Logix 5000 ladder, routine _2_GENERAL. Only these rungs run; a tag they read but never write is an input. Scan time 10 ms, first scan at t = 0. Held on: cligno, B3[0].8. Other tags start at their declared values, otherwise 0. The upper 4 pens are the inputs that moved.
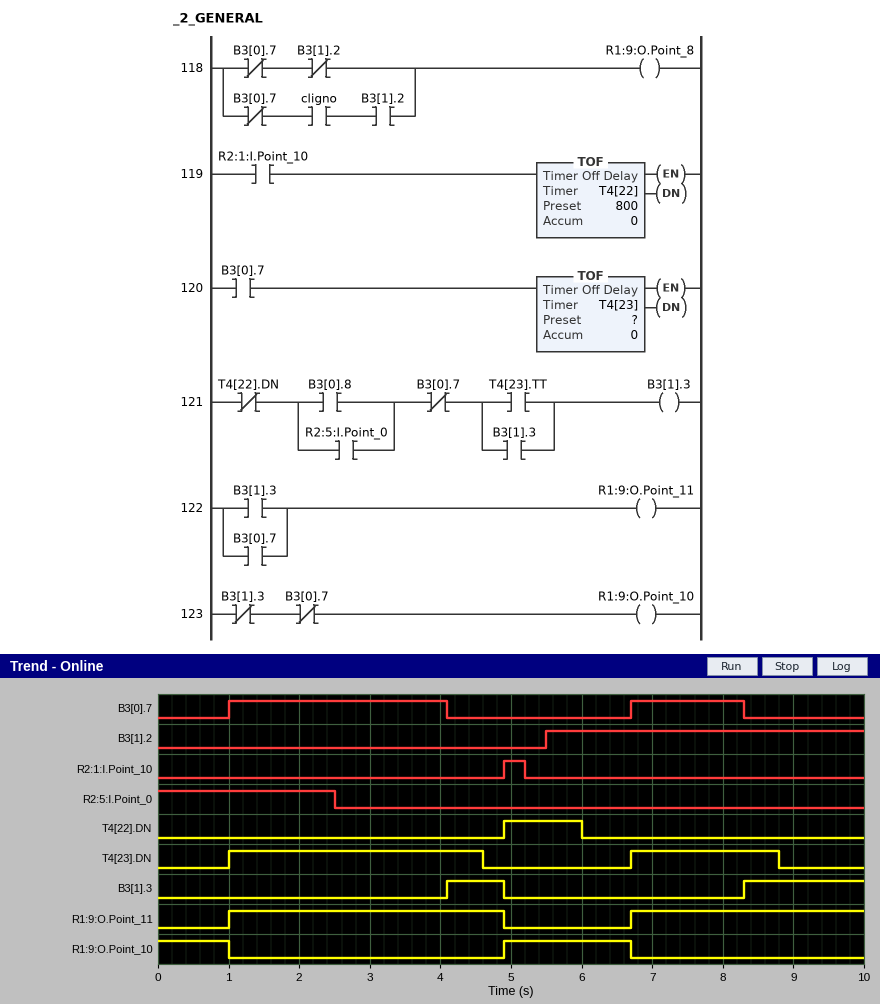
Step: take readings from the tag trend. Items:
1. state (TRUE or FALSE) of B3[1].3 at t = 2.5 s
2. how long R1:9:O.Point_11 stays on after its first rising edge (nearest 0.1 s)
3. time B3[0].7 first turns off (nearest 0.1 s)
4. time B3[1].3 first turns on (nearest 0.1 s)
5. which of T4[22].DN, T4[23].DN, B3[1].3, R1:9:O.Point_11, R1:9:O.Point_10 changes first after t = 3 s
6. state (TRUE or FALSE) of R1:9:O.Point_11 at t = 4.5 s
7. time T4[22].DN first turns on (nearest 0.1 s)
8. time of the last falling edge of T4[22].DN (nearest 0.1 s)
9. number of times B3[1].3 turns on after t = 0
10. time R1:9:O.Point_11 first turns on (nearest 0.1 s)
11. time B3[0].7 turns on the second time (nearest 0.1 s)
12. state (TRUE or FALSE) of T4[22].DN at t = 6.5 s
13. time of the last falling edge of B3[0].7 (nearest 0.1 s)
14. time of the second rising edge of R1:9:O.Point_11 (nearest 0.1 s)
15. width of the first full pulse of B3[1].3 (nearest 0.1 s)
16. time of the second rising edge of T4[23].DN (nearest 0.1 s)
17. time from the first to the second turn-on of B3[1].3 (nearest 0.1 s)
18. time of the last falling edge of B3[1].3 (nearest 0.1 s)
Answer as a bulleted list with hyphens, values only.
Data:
- FALSE
- 3.9 s
- 4.1 s
- 4.1 s
- B3[1].3
- TRUE
- 4.9 s
- 6.0 s
- 2
- 1.0 s
- 6.7 s
- FALSE
- 8.3 s
- 6.7 s
- 0.8 s
- 6.7 s
- 4.2 s
- 4.9 s
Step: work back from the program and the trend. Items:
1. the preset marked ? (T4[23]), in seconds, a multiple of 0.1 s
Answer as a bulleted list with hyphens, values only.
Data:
- 0.5 s
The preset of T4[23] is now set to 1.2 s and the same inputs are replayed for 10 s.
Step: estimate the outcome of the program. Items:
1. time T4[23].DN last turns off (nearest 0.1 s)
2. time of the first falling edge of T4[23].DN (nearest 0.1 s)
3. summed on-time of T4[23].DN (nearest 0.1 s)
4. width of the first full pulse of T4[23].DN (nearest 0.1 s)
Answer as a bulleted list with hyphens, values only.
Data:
- 9.5 s
- 5.3 s
- 7.1 s
- 4.3 s
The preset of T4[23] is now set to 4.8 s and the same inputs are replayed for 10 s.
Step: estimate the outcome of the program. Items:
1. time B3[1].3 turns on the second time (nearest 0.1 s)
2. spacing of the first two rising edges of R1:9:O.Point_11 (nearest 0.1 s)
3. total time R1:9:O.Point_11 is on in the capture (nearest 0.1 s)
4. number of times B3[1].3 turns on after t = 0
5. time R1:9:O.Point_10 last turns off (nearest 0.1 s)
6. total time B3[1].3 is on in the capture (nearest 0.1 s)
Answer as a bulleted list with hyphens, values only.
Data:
- 6.0 s
- 5.0 s
- 7.9 s
- 3
- 6.0 s
- 3.2 s
